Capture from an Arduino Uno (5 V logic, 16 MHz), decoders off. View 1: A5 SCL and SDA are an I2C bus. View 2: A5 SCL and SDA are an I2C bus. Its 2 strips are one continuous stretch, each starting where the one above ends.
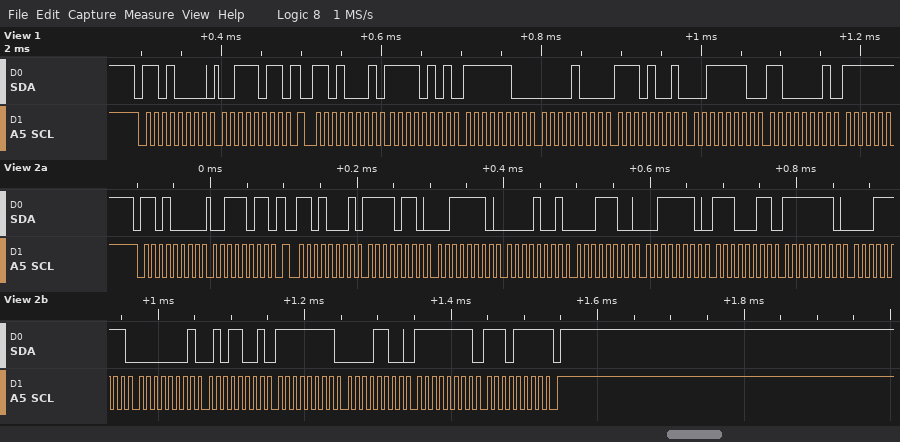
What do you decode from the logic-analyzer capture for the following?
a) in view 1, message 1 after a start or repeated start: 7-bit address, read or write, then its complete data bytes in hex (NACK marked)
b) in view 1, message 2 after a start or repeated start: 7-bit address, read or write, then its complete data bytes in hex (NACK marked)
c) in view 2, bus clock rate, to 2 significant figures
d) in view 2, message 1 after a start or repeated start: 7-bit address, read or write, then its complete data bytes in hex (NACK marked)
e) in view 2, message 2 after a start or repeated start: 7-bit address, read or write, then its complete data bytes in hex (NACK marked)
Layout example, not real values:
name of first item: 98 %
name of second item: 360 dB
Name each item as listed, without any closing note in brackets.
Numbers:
in view 1, message 1 after a start or repeated start: 7-bit address, read or write, then its complete data bytes in hex: 0x68 write: 3B
in view 1, message 2 after a start or repeated start: 7-bit address, read or write, then its complete data bytes in hex: 0x68 read: F5 FC 08 E9 3E C1
in view 2, bus clock rate, to 2 significant figures: 100 kHz
in view 2, message 1 after a start or repeated start: 7-bit address, read or write, then its complete data bytes in hex: 0x68 write: 3B
in view 2, message 2 after a start or repeated start: 7-bit address, read or write, then its complete data bytes in hex: 0x68 read: F6 3E 09 1C 3E E3 FE 1F 01 59 FF 0C FF EF NACK
